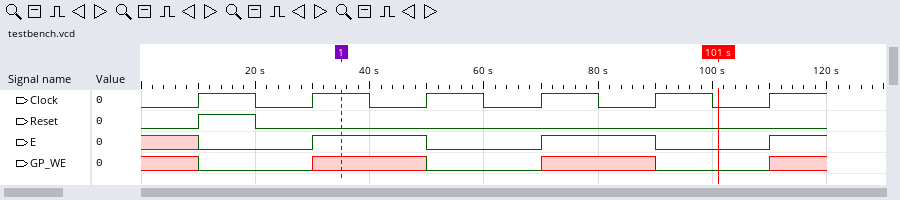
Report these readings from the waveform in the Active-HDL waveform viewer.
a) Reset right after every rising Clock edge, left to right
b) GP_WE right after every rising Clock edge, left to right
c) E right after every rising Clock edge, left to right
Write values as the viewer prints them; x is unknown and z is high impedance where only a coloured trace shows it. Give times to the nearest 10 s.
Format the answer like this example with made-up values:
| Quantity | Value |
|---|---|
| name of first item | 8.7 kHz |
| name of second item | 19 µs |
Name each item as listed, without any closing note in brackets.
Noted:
| Quantity | Value |
|---|---|
| Reset right after every rising Clock edge, left to right | 1 0 0 0 0 0 |
| GP_WE right after every rising Clock edge, left to right | 0 x 0 x 0 x |
| E right after every rising Clock edge, left to right | 0 1 0 1 0 1 |
